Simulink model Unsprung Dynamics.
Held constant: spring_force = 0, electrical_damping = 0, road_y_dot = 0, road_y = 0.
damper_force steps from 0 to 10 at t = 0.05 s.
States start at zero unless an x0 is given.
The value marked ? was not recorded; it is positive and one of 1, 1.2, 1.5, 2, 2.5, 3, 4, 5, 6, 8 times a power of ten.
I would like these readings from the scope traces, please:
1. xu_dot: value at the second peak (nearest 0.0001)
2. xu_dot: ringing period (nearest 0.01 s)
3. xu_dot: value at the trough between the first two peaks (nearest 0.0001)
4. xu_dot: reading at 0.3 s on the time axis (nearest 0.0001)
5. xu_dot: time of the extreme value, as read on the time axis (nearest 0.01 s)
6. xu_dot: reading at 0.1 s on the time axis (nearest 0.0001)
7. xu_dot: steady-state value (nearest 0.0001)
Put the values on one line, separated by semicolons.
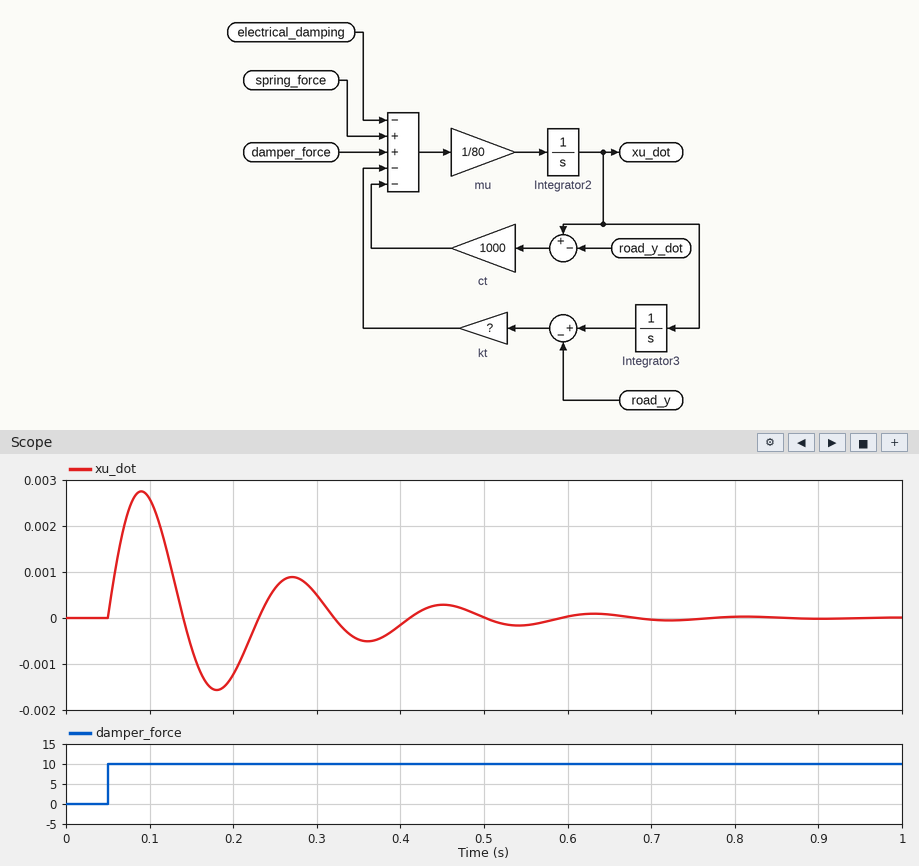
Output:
0.0009; 0.18 s; -0.0016; 0.0005; 0.09 s; 0.0026; 0.0000
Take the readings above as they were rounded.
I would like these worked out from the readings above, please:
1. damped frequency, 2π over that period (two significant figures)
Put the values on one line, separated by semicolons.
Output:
35 rad/s
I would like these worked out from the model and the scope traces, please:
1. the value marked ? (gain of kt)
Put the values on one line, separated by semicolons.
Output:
100000
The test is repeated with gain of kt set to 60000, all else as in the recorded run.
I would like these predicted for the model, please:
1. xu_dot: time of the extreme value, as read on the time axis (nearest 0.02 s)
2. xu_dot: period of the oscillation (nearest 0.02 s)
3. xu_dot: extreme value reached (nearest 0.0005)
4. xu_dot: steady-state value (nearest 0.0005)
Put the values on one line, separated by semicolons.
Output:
0.10 s; 0.24 s; 0.0035; 0.0000
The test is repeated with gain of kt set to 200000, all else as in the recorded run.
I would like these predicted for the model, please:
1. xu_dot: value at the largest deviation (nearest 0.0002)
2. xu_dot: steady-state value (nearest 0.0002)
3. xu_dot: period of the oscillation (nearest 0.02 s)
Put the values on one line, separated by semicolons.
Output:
0.0020; 0.0000; 0.12 s
